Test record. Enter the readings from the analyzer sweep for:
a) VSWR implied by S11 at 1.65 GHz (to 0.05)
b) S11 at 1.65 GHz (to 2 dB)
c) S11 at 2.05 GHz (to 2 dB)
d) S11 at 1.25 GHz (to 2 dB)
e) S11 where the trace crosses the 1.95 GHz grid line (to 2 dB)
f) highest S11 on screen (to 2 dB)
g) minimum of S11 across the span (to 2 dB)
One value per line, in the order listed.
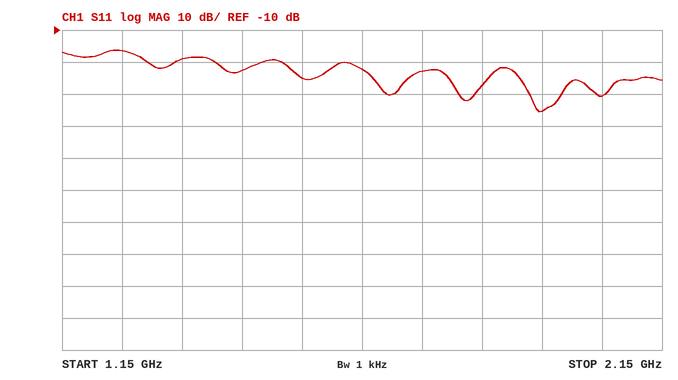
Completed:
1.15
-22 dB
-30 dB
-16 dB
-36 dB
-16 dB
-36 dB
